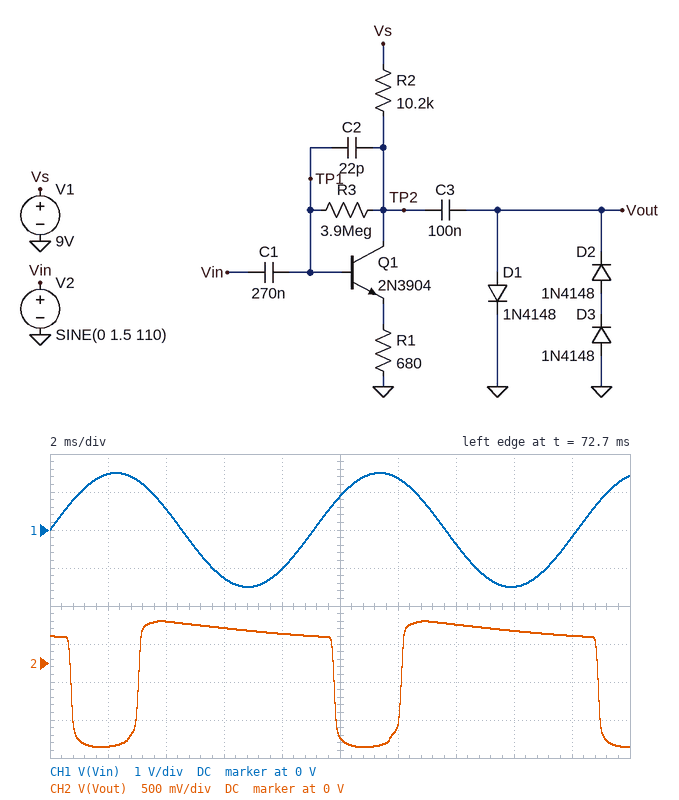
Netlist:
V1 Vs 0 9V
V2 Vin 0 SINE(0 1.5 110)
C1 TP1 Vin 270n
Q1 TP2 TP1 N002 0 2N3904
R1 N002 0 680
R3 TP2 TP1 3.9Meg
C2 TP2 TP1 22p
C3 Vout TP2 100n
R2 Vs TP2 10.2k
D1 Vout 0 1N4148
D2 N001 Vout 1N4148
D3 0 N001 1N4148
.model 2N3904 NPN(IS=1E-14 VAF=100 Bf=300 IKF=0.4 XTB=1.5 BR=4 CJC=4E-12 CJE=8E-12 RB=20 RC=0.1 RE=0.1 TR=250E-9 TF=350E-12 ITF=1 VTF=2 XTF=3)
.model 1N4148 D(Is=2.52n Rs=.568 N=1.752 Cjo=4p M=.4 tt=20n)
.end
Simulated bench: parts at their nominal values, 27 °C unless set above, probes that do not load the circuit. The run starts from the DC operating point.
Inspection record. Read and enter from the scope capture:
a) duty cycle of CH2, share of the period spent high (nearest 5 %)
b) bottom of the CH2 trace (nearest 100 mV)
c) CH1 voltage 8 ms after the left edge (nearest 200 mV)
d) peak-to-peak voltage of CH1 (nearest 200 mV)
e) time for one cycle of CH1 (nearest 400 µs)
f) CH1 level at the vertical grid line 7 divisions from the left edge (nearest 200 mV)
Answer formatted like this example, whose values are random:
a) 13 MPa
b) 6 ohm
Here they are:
a) 75 %
b) -1.1 V
c) -1.0 V
d) 3.0 V
e) 9.2 ms
f) -400 mV
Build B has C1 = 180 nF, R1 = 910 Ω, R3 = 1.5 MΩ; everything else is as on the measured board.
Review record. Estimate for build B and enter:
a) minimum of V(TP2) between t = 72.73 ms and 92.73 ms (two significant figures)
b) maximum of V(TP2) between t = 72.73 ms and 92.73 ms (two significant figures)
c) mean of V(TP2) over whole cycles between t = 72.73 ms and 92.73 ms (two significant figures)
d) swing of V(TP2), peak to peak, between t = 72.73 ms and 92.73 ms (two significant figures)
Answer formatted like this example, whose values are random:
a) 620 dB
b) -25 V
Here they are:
a) 850 mV
b) 8.9 V
c) 6.3 V
d) 8.0 V
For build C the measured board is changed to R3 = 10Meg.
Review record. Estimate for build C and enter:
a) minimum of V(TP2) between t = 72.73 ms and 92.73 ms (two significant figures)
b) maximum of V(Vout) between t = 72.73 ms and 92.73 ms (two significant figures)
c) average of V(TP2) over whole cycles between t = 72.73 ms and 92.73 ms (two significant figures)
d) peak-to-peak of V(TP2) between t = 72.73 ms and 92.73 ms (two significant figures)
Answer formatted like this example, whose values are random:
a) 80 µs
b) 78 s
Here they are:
a) 2.0 V
b) 540 mV
c) 7.1 V
d) 6.9 V
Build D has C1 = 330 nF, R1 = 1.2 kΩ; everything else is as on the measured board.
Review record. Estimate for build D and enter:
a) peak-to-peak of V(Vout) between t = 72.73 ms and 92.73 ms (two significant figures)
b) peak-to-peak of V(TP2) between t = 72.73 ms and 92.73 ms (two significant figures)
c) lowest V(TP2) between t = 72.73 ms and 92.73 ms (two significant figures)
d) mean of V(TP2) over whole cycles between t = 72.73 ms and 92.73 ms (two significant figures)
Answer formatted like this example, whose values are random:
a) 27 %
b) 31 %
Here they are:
a) 1.6 V
b) 7.8 V
c) 1.1 V
d) 6.2 V
